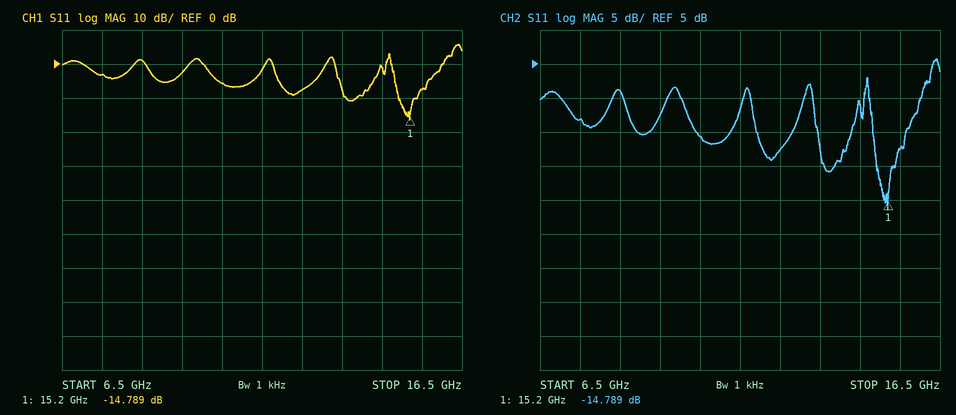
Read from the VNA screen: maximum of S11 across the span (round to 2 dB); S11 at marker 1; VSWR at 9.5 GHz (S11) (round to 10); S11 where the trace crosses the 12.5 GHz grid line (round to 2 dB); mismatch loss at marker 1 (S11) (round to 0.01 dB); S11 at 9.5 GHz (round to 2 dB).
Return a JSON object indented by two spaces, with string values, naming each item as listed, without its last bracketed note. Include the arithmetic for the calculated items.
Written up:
{
  "maximum of S11 across the span": "6 dB",
  "S11 at marker 1": "-14.789 dB",
  "VSWR at 9.5 GHz (S11)": "|Γ| = 10^(-2/20) = 0.7943; VSWR = (1 + 0.7943)/(1 − 0.7943) ≈ 8.72, so 10 to the nearest 10",
  "S11 where the trace crosses the 12.5 GHz grid line": "-8 dB",
  "mismatch loss at marker 1 (S11)": "−10 log10(1 − 10^(-14.789/10)) ≈ 0.15 dB",
  "S11 at 9.5 GHz": "-2 dB"
}
